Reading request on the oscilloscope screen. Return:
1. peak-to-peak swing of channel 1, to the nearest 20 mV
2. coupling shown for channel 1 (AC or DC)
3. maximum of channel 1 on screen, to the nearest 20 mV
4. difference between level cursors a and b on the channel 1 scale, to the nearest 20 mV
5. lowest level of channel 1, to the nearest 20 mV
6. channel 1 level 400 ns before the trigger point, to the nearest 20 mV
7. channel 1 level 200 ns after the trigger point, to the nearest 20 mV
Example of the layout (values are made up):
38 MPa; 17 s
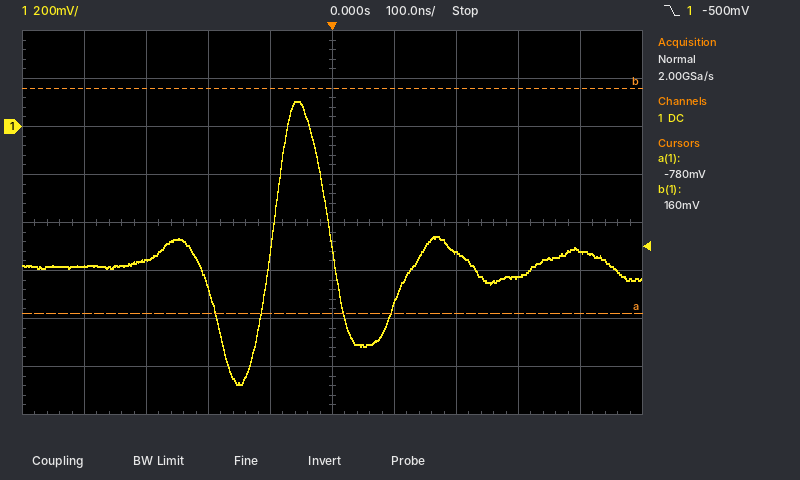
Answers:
1.18 V; DC; 100 mV; 940 mV; -1.08 V; -580 mV; -520 mV
